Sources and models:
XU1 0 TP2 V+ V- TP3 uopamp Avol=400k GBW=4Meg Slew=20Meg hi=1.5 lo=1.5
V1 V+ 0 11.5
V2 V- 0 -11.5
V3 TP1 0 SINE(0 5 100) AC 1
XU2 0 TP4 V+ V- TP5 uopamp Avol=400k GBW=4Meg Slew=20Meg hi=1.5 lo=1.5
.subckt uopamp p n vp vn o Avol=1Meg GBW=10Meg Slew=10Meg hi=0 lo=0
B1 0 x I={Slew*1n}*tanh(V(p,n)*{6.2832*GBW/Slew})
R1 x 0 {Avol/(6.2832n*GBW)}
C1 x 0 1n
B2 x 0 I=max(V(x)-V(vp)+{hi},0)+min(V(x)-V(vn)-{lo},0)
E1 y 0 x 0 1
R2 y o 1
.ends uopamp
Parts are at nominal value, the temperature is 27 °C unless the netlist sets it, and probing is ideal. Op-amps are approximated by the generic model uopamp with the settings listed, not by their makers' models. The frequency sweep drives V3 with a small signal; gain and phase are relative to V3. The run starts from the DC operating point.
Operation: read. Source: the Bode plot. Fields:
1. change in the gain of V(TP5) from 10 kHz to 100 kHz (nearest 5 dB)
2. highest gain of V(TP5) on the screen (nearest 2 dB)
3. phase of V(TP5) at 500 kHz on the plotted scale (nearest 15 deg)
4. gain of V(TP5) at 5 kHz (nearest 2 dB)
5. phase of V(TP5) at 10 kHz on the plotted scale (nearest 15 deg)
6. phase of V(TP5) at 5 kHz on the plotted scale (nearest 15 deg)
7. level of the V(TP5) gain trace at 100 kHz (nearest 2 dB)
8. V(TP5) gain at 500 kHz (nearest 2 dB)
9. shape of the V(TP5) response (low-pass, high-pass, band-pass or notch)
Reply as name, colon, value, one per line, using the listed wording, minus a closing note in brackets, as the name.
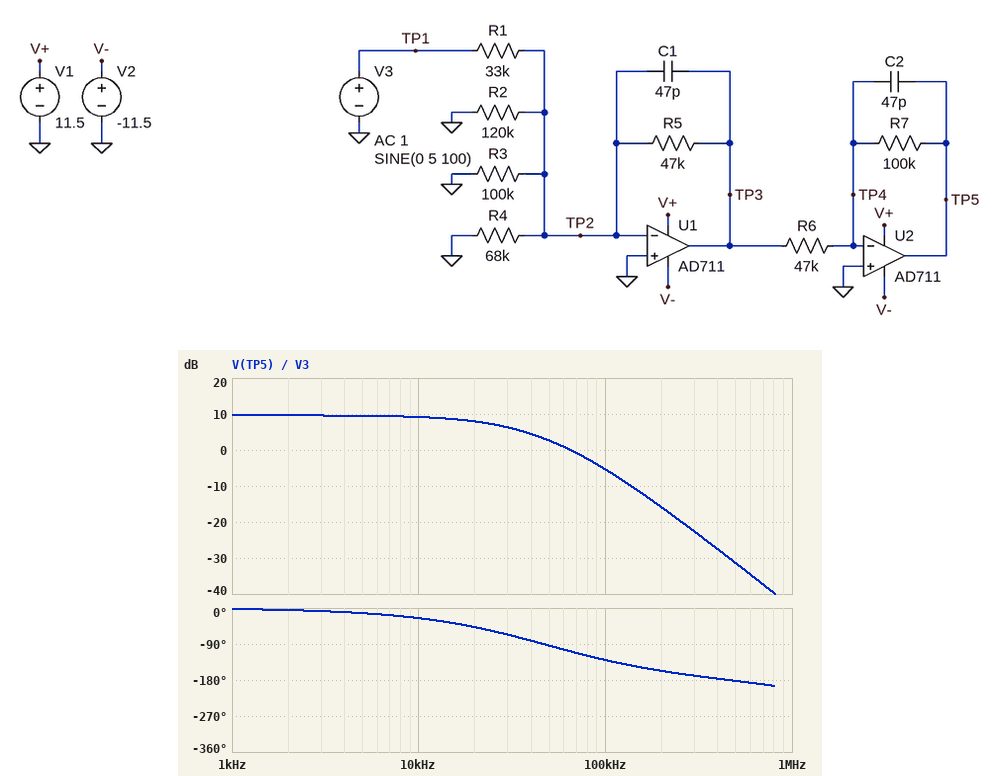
change in the gain of V(TP5) from 10 kHz to 100 kHz: -15 dB
highest gain of V(TP5) on the screen: 10 dB
phase of V(TP5) at 500 kHz on the plotted scale: -180 deg
gain of V(TP5) at 5 kHz: 10 dB
phase of V(TP5) at 10 kHz on the plotted scale: -30 deg
phase of V(TP5) at 5 kHz on the plotted scale: -15 deg
level of the V(TP5) gain trace at 100 kHz: -6 dB
V(TP5) gain at 500 kHz: -32 dB
shape of the V(TP5) response: low-pass
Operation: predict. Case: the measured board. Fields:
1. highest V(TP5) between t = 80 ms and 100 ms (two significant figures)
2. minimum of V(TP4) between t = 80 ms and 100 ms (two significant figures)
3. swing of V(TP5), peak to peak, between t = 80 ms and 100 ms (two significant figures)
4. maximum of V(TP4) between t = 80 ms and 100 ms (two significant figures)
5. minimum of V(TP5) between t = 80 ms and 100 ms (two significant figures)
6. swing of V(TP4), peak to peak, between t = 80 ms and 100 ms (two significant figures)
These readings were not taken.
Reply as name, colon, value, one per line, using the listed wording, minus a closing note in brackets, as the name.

highest V(TP5) between t = 80 ms and 100 ms: 10 V
minimum of V(TP4) between t = 80 ms and 100 ms: -1.6 V
swing of V(TP5), peak to peak, between t = 80 ms and 100 ms: 20 V
maximum of V(TP4) between t = 80 ms and 100 ms: 1.6 V
minimum of V(TP5) between t = 80 ms and 100 ms: -10 V
swing of V(TP4), peak to peak, between t = 80 ms and 100 ms: 3.3 V
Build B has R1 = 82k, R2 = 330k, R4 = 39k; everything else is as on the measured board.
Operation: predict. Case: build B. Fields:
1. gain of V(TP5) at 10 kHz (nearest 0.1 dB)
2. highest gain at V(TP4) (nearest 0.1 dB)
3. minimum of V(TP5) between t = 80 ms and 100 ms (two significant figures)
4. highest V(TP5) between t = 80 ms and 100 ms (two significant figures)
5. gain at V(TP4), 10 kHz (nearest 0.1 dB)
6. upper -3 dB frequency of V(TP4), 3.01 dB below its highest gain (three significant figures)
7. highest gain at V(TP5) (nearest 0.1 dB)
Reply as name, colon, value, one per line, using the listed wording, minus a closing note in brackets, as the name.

gain of V(TP5) at 10 kHz: 1.3 dB
highest gain at V(TP4): -43.3 dB
minimum of V(TP5) between t = 80 ms and 100 ms: -6.1 V
highest V(TP5) between t = 80 ms and 100 ms: 6.1 V
gain at V(TP4), 10 kHz: -50.8 dB
upper -3 dB frequency of V(TP4), 3.01 dB below its highest gain: 121 kHz
highest gain at V(TP5): 1.7 dB
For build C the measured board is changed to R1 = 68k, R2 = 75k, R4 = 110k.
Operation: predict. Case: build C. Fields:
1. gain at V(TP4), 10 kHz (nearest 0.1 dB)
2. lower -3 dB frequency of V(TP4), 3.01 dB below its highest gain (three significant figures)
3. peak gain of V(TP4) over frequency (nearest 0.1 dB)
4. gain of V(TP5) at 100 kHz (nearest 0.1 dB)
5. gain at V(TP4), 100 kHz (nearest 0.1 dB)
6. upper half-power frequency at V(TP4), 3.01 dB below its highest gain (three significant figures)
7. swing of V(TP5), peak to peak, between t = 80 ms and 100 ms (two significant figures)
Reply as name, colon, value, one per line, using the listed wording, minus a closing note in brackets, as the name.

gain at V(TP4), 10 kHz: -49.2 dB
lower -3 dB frequency of V(TP4), 3.01 dB below its highest gain: 19.0 kHz
peak gain of V(TP4) over frequency: -41.7 dB
gain of V(TP5) at 100 kHz: -11.6 dB
gain at V(TP4), 100 kHz: -43.6 dB
upper half-power frequency at V(TP4), 3.01 dB below its highest gain: 121 kHz
swing of V(TP5), peak to peak, between t = 80 ms and 100 ms: 15 V
